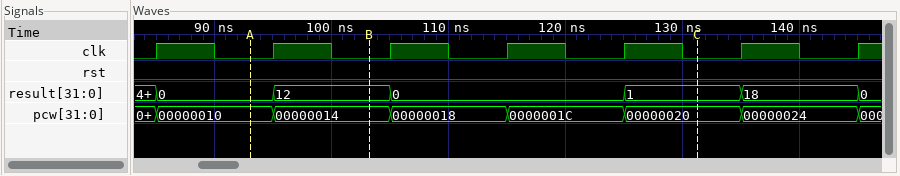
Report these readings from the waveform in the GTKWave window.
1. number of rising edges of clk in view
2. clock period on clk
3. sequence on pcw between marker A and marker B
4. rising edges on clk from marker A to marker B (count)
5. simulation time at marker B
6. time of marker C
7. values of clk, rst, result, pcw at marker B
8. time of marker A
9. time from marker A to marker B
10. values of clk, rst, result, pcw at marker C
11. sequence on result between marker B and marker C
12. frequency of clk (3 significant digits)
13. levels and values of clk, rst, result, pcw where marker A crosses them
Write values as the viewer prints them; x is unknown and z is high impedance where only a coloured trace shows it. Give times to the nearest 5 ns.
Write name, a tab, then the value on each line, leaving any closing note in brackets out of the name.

number of rising edges of clk in view	7
clock period on clk	10 ns
sequence on pcw between marker A and marker B	00000010, 00000014
rising edges on clk from marker A to marker B	1
simulation time at marker B	105 ns
time of marker C	130 ns
values of clk, rst, result, pcw at marker B	clk=0, rst=0, result=12, pcw=00000014
time of marker A	95 ns
time from marker A to marker B	10 ns
values of clk, rst, result, pcw at marker C	clk=0, rst=0, result=1, pcw=00000020
sequence on result between marker B and marker C	12, 0, 1
frequency of clk	100 MHz
levels and values of clk, rst, result, pcw where marker A crosses them	clk=0, rst=0, result=0, pcw=00000010
